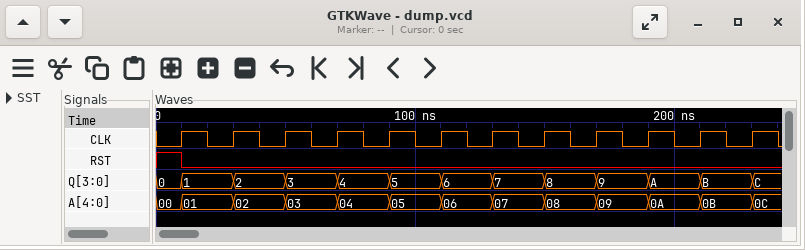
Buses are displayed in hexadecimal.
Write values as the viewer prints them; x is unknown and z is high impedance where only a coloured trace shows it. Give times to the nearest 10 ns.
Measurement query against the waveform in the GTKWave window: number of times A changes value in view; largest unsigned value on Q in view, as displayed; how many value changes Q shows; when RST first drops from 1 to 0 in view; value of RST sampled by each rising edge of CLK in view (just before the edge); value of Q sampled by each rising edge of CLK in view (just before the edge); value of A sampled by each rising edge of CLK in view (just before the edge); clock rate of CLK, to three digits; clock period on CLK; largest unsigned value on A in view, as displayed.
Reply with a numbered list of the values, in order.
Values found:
1. 12
2. C
3. 12
4. 10 ns
5. 1 0 0 0 0 0 0 0 0 0 0 0
6. 0, 1, 2, 3, 4, 5, 6, 7, 8, 9, A, B
7. 00, 01, 02, 03, 04, 05, 06, 07, 08, 09, 0A, 0B
8. 50.0 MHz
9. 20 ns
10. 0C
